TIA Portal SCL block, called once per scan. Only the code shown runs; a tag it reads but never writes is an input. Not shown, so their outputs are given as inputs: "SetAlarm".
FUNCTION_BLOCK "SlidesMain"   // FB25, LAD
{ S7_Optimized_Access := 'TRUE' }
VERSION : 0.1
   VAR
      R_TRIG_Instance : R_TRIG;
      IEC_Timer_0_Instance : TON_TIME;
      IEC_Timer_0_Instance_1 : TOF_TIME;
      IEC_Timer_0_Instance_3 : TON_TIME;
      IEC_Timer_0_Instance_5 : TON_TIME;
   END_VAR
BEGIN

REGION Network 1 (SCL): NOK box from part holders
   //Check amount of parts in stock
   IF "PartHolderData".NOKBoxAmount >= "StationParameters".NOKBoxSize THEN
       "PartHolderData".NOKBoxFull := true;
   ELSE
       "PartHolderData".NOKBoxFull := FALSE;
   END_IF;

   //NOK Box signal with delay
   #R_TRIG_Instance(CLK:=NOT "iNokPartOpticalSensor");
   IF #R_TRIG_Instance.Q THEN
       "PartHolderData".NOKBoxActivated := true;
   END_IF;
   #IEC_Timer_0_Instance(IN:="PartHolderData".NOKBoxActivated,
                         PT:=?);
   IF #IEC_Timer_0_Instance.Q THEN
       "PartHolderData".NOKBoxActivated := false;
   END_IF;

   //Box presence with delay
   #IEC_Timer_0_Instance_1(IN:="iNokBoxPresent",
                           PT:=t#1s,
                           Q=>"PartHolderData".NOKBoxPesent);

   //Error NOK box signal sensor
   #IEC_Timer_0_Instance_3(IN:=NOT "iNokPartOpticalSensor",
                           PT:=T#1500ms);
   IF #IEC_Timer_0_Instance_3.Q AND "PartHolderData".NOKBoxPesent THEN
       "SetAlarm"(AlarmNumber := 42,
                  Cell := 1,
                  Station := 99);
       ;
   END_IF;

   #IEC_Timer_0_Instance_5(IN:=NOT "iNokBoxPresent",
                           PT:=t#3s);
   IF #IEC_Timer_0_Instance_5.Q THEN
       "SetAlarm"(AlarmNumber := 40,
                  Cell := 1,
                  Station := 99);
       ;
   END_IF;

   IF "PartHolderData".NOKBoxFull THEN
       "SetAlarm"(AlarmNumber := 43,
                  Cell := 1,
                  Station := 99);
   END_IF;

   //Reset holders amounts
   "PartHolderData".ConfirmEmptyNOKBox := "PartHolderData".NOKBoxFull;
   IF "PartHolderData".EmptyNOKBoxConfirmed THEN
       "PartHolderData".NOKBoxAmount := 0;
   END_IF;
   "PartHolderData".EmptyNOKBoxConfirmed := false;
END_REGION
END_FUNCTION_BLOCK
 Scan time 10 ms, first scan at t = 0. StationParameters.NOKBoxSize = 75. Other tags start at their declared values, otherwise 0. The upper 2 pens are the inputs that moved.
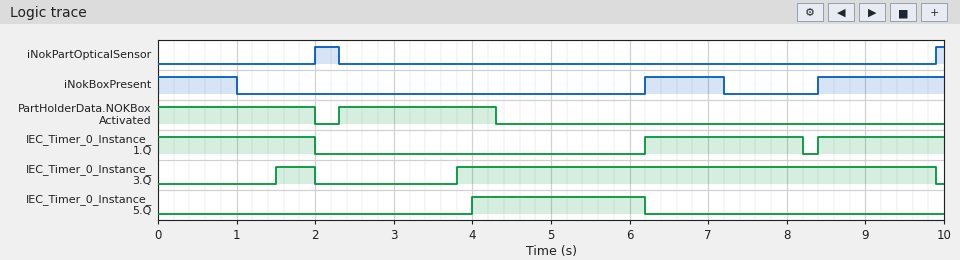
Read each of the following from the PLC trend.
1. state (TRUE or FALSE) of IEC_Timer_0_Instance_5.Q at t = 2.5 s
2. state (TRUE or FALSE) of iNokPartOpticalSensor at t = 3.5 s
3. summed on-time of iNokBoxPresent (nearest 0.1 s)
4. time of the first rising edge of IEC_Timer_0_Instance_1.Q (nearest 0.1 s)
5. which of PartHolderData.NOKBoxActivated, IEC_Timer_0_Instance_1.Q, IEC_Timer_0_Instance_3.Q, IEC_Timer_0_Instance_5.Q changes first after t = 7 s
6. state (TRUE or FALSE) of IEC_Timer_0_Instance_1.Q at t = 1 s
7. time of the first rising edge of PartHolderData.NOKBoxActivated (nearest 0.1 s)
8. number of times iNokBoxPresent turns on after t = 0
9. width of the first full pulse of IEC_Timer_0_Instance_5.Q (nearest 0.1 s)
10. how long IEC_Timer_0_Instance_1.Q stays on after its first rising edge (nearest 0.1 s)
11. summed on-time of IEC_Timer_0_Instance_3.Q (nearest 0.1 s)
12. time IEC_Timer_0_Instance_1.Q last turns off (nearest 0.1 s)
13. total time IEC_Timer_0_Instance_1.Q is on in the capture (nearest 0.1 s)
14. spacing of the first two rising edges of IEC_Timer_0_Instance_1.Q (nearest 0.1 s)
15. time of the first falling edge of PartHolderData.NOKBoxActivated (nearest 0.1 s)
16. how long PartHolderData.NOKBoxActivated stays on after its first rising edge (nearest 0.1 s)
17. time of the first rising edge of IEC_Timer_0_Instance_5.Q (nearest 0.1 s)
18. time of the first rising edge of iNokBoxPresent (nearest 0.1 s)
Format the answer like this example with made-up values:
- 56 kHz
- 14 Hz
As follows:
- FALSE
- FALSE
- 3.6 s
- 6.2 s
- IEC_Timer_0_Instance_1.Q
- TRUE
- 2.3 s
- 2
- 2.2 s
- 2.0 s
- 6.6 s
- 8.2 s
- 5.6 s
- 2.2 s
- 2.0 s
- 2.0 s
- 4.0 s
- 6.2 s
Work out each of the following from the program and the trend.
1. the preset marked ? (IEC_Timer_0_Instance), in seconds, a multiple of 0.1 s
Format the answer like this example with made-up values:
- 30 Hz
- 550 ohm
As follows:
- 2.0 s
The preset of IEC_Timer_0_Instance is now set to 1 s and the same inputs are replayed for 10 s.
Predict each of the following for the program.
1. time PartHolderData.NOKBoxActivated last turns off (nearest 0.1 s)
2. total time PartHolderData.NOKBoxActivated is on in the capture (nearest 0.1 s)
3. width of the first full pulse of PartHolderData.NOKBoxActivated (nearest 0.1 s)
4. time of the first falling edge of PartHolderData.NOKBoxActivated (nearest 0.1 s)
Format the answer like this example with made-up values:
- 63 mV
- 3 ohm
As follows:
- 3.3 s
- 2.0 s
- 1.0 s
- 1.0 s
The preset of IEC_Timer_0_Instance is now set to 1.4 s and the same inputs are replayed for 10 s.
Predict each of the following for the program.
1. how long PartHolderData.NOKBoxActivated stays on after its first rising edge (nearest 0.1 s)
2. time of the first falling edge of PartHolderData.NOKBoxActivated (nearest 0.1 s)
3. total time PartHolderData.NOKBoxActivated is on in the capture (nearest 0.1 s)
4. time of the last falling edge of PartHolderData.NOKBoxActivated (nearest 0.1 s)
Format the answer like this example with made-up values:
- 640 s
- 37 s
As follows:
- 1.4 s
- 1.4 s
- 2.8 s
- 3.7 s
